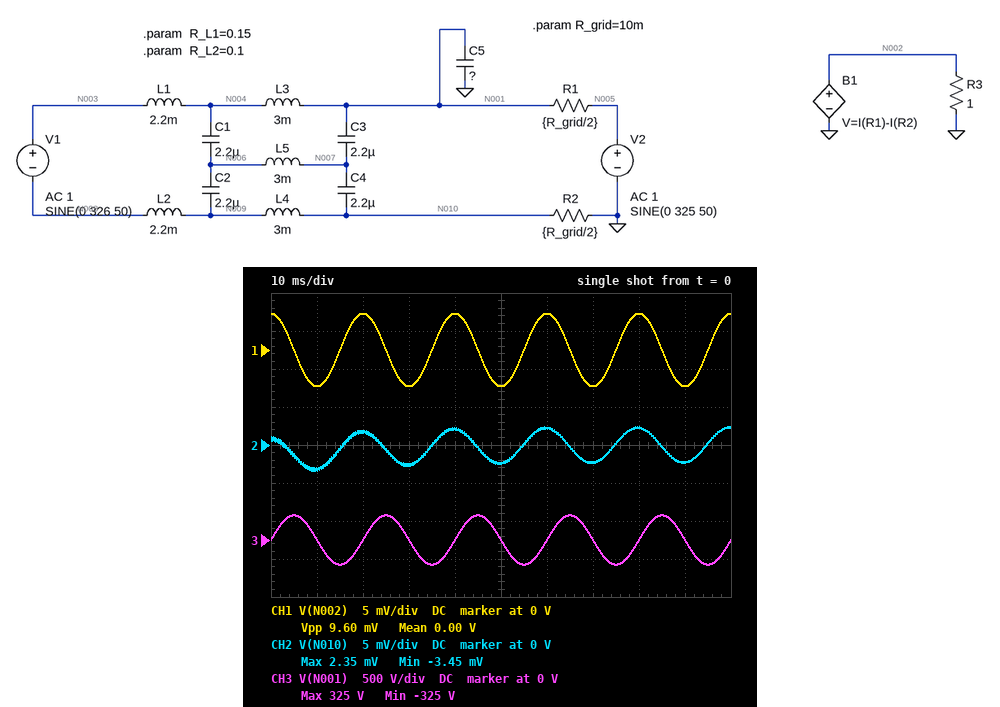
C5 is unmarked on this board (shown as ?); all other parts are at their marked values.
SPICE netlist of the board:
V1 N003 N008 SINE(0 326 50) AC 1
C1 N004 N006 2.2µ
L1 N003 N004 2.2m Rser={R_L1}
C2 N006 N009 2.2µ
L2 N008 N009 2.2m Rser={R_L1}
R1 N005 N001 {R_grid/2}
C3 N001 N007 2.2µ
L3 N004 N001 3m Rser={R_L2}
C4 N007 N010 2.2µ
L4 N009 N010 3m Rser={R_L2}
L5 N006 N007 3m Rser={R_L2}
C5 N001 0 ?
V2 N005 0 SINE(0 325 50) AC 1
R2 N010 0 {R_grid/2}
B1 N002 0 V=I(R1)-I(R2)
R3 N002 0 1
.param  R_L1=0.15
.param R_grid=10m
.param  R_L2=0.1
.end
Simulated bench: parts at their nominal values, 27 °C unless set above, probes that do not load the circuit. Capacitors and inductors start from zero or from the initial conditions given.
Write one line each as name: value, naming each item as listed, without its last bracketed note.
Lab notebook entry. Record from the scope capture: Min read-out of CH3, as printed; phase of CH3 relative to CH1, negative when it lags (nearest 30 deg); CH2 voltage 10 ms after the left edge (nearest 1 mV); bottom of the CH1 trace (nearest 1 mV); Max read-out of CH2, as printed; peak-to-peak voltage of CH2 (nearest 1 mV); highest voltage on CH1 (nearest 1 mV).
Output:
Min read-out of CH3, as printed: -325 V
phase of CH3 relative to CH1, negative when it lags: -90 deg
CH2 voltage 10 ms after the left edge: -3 mV
bottom of the CH1 trace: -5 mV
Max read-out of CH2, as printed: 2.35 mV
peak-to-peak voltage of CH2: 6 mV
highest voltage on CH1: 5 mV
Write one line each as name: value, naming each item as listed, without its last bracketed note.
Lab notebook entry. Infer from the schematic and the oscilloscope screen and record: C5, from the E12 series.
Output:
C5, from the E12 series: 47 nF
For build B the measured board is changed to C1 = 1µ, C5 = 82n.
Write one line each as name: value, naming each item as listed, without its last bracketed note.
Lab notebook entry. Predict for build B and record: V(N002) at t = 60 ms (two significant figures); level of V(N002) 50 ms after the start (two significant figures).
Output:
V(N002) at t = 60 ms: 8.4 mV
level of V(N002) 50 ms after the start: -8.4 mV
